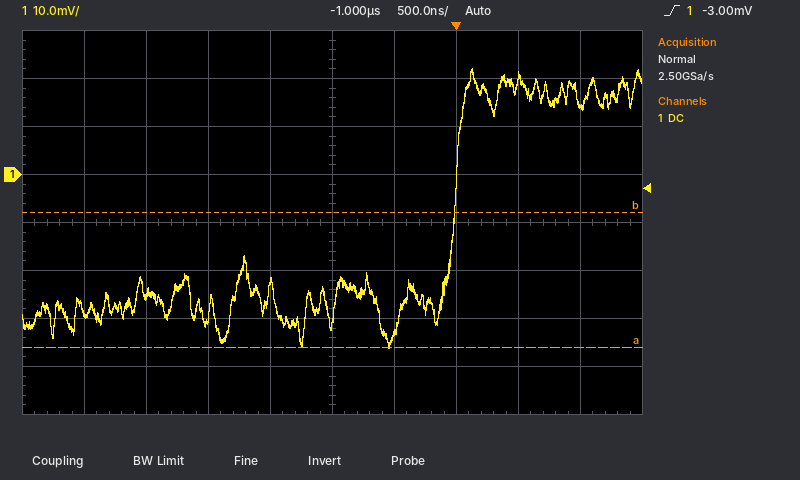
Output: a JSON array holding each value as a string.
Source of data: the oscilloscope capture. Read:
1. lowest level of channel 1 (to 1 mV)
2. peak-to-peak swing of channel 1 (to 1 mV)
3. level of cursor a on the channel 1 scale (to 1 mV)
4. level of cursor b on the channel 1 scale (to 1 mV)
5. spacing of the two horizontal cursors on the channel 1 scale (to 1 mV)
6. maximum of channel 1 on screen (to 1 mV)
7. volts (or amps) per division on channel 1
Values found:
["-36 mV", "58 mV", "-36 mV", "-8 mV", "28 mV", "22 mV", "10 mV"]
